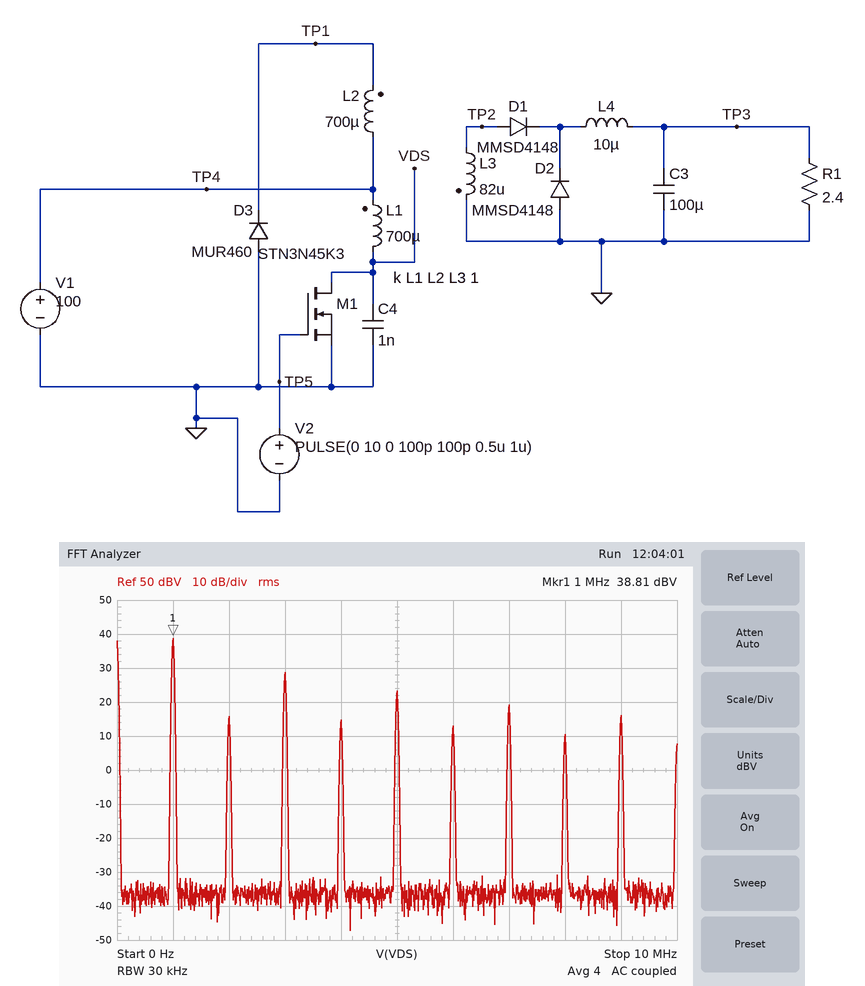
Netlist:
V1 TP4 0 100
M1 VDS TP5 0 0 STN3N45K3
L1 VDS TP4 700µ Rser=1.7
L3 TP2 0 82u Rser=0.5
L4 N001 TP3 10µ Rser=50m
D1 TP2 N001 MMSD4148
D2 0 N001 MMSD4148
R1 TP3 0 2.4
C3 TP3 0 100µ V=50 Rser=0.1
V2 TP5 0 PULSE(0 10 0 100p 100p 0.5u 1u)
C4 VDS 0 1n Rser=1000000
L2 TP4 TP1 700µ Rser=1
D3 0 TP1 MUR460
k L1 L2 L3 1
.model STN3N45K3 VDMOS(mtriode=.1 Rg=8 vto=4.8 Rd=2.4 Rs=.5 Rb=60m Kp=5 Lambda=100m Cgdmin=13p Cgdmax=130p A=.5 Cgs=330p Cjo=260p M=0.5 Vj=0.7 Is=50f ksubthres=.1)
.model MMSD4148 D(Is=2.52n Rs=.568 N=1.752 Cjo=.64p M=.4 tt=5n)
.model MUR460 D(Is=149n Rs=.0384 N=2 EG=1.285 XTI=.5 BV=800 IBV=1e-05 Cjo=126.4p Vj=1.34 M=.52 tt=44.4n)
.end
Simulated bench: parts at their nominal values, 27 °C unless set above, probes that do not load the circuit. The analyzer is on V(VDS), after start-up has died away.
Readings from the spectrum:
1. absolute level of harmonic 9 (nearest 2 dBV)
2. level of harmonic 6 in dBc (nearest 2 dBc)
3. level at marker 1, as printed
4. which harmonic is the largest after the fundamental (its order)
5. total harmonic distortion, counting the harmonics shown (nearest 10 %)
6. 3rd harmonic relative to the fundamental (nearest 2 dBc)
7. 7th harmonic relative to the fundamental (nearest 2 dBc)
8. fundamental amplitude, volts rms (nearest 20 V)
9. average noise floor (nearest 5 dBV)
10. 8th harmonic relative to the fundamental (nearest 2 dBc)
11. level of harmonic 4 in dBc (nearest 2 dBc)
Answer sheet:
16 dBV
-26 dBc
38.81 dBV
3
40 %
-10 dBc
-20 dBc
80 V
-35 dBV
-28 dBc
-24 dBc
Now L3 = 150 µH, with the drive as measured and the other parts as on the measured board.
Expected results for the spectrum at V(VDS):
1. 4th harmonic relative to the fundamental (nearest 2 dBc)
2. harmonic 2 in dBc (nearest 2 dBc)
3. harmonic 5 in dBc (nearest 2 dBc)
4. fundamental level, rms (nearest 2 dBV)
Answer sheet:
-20 dBc
-18 dBc
-18 dBc
38 dBV
